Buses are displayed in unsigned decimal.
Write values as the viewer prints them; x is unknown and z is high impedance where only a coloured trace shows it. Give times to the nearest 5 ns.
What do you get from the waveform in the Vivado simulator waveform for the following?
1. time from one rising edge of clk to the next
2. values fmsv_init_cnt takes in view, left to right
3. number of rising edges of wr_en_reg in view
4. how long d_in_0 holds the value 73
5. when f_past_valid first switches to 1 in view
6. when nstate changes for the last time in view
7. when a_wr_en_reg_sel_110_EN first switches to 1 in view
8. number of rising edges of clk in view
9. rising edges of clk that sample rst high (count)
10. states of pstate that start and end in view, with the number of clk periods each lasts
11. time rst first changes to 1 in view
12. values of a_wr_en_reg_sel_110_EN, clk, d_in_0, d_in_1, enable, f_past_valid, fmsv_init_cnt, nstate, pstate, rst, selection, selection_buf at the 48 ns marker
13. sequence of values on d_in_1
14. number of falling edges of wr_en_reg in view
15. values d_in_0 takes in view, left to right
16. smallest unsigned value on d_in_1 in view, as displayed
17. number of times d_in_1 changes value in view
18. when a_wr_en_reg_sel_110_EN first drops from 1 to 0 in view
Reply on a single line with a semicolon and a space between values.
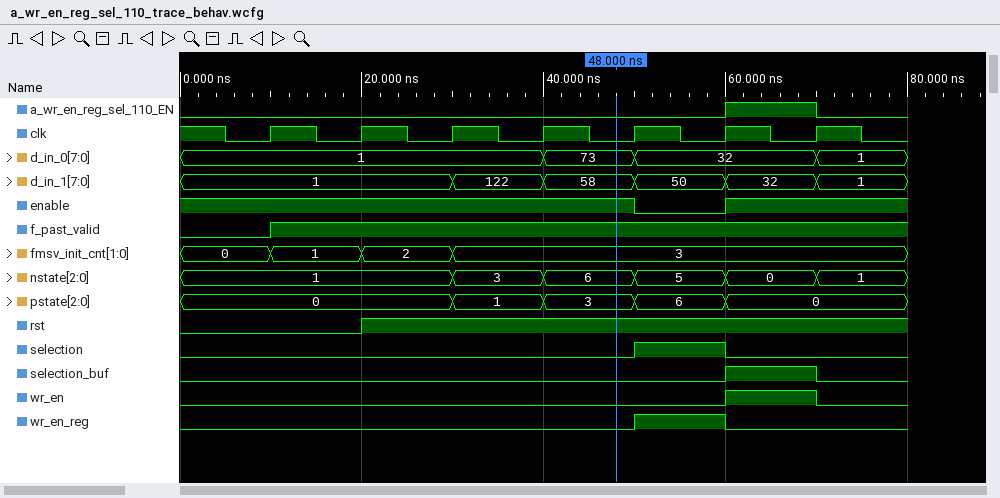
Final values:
10 ns; 0, 1, 2, 3; 1; 10 ns; 10 ns; 70 ns; 60 ns; 7; 5; 1: 1, 3: 1, 6: 1; 20 ns; a_wr_en_reg_sel_110_EN=0, clk=0, d_in_0=73, d_in_1=58, enable=1, f_past_valid=1, fmsv_init_cnt=3, nstate=6, pstate=3, rst=1, selection=0, selection_buf=0; 1, 122, 58, 50, 32, 1; 1; 1, 73, 32, 1; 1; 5; 70 ns
